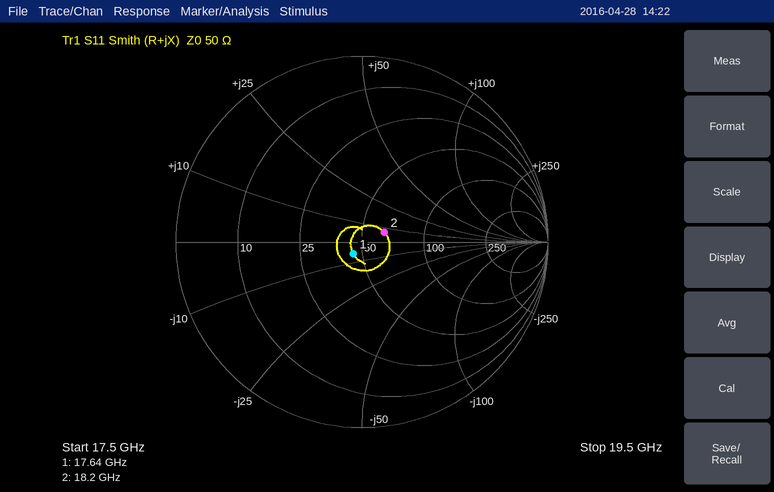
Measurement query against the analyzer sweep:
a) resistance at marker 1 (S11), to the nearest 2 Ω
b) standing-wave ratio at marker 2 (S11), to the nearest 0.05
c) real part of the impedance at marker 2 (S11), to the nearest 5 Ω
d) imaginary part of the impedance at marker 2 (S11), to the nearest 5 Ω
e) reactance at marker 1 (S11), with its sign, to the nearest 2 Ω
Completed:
46 Ω
1.30
65 Ω
+5 Ω
-6 Ω
